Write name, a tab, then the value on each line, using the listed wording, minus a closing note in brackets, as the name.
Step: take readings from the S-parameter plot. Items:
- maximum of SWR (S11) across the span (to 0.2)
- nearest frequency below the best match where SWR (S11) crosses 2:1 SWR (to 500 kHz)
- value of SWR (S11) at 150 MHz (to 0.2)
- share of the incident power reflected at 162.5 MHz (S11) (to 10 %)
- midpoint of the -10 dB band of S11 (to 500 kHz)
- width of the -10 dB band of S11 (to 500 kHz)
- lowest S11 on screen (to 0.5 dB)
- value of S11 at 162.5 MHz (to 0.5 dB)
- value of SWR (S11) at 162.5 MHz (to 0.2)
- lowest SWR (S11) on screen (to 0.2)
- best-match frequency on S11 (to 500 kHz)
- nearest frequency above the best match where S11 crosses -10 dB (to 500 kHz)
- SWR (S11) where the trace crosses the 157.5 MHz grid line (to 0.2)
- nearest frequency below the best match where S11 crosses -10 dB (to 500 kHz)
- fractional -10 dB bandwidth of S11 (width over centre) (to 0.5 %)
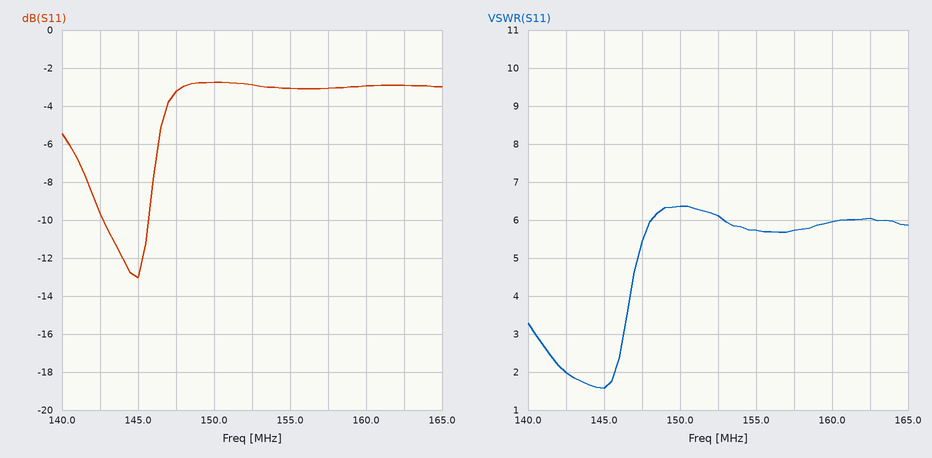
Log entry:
maximum of SWR (S11) across the span	6.4
nearest frequency below the best match where SWR (S11) crosses 2:1 SWR	142.5 MHz
value of SWR (S11) at 150 MHz	6.4
share of the incident power reflected at 162.5 MHz (S11)	50 %
midpoint of the -10 dB band of S11	144.0 MHz
width of the -10 dB band of S11	3.0 MHz
lowest S11 on screen	-13.0 dB
value of S11 at 162.5 MHz	-3.0 dB
value of SWR (S11) at 162.5 MHz	6.0
lowest SWR (S11) on screen	1.6
best-match frequency on S11	145.0 MHz
nearest frequency above the best match where S11 crosses -10 dB	145.5 MHz
SWR (S11) where the trace crosses the 157.5 MHz grid line	5.8
nearest frequency below the best match where S11 crosses -10 dB	142.5 MHz
fractional -10 dB bandwidth of S11 (width over centre)	2.0 %
